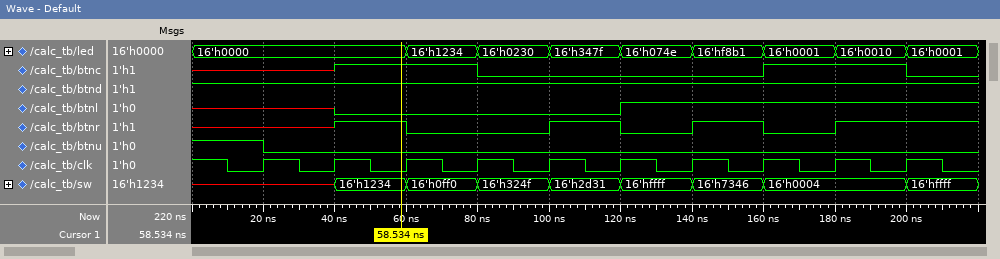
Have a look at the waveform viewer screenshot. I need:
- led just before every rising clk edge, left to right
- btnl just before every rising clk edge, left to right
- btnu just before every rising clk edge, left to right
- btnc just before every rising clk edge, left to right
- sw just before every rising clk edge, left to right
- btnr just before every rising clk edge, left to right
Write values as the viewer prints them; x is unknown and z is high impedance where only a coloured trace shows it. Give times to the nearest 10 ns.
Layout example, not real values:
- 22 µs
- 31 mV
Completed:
- 16'h0000, 16'h0000, 16'h0000, 16'h1234, 16'h0230, 16'h347f, 16'h074e, 16'hf8b1, 16'h0001, 16'h0010
- x x 0 0 0 0 1 1 1 1
- 1 0 0 0 0 0 0 0 0 0
- x x 1 1 0 0 0 0 1 1
- x, x, 16'h1234, 16'h0ff0, 16'h324f, 16'h2d31, 16'hffff, 16'h7346, 16'h0004, 16'h0004
- x x 1 0 0 1 0 1 0 1
